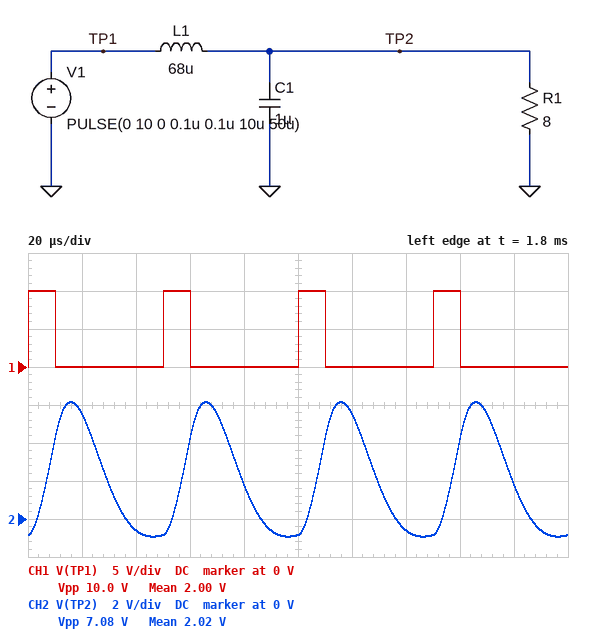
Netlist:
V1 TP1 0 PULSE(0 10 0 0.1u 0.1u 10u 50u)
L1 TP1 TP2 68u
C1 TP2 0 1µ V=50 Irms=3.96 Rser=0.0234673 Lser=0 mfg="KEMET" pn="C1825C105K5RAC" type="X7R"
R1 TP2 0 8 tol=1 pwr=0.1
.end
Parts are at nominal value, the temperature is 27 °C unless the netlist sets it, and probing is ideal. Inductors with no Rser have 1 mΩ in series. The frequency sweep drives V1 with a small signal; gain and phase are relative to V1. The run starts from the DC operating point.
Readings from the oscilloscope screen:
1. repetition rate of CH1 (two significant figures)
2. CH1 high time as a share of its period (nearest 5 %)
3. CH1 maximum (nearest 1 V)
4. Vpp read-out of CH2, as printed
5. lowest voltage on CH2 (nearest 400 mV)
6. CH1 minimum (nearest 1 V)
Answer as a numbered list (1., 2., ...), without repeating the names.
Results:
1. 20 kHz
2. 20 %
3. 10 V
4. 7.08 V
5. -800 mV
6. 0 V
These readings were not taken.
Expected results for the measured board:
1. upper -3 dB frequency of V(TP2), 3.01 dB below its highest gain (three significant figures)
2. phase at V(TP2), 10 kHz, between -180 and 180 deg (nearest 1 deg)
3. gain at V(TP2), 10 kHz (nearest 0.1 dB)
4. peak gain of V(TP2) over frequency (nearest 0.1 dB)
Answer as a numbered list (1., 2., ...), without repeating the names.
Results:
1. 22.4 kHz
2. -36 deg
3. 0.9 dB
4. 1.1 dB
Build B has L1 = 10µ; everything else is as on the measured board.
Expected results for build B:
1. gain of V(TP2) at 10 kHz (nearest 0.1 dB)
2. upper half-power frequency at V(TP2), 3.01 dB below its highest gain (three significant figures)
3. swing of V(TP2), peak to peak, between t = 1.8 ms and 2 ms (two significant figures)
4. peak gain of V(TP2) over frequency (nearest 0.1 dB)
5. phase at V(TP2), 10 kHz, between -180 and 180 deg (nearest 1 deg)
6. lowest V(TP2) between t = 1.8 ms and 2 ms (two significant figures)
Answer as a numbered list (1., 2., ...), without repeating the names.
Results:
1. 0.3 dB
2. 57.6 kHz
3. 22 V
4. 8.1 dB
5. -5 deg
6. -7.7 V
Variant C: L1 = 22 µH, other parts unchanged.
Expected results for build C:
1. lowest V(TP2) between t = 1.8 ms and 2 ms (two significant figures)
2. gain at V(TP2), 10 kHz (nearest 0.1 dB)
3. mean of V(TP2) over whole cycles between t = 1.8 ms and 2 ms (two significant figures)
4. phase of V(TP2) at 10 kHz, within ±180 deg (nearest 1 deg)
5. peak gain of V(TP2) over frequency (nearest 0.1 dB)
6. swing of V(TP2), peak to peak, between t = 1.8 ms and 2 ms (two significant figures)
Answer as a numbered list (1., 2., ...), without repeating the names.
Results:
1. -4.3 V
2. 0.6 dB
3. 2.0 V
4. -11 deg
5. 5.0 dB
6. 16 V
